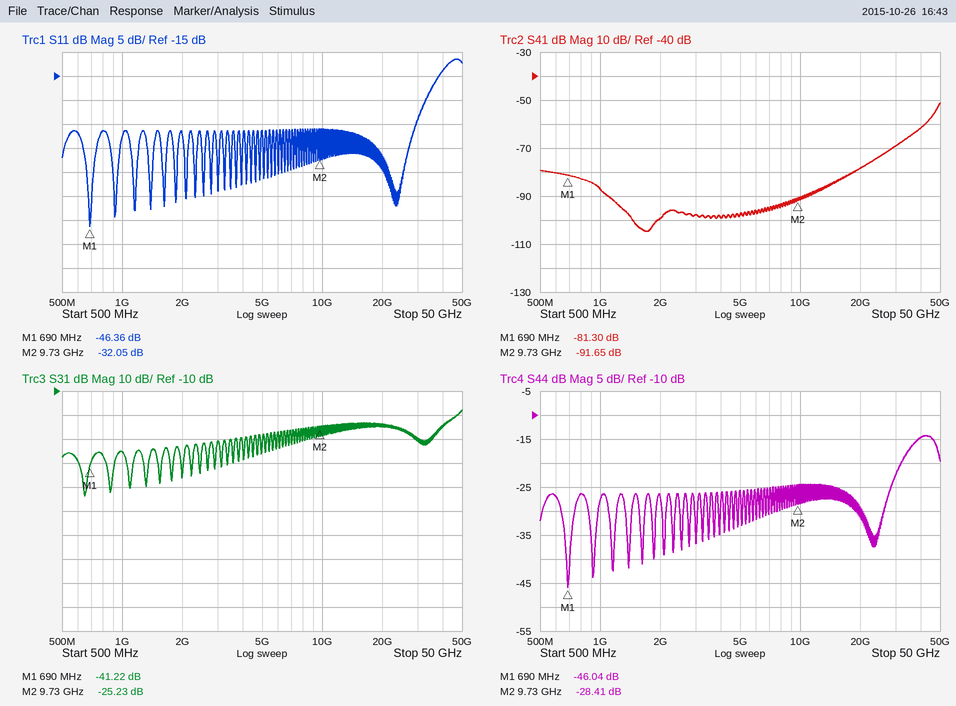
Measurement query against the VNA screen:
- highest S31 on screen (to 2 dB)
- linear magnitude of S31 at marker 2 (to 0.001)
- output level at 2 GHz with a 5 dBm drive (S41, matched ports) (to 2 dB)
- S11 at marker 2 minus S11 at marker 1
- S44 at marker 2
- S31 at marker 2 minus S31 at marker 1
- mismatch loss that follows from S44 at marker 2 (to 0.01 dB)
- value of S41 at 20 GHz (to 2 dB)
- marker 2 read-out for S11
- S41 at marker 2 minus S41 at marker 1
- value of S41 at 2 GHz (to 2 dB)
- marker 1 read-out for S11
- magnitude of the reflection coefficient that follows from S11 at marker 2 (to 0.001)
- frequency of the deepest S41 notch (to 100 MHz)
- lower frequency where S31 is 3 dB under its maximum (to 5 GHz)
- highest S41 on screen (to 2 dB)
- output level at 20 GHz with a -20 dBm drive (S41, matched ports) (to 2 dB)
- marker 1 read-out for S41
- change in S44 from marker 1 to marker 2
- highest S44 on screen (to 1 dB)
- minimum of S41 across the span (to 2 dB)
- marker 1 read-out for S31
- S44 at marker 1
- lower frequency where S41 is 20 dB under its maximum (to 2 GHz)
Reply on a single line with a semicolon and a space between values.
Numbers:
-18 dB; 0.055; -94 dBm; 14.31 dB; -28.41 dB; 15.99 dB; 0.01 dB; -78 dB; -32.05 dB; -10.35 dB; -100 dB; -46.36 dB; 0.025; 1.7 GHz; 45 GHz; -52 dB; -98 dBm; -81.30 dB; 17.63 dB; -14 dB; -104 dB; -41.22 dB; -46.04 dB; 28 GHz
